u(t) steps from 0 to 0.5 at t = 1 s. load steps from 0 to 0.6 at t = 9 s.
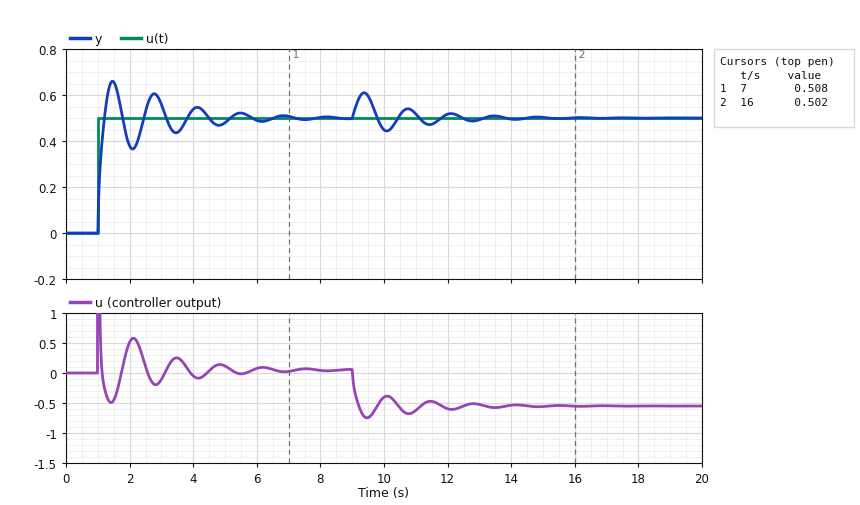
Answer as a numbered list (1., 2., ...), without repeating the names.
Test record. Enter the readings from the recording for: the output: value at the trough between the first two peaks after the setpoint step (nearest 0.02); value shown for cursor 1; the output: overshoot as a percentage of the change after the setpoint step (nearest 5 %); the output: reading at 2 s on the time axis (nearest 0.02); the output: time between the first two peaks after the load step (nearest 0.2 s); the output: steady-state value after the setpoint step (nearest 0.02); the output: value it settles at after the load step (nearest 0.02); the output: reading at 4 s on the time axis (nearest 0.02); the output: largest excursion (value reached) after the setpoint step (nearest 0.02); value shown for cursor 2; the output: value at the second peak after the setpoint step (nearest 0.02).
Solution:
1. 0.36
2. 0.508
3. 30 %
4. 0.38
5. 1.4 s
6. 0.50
7. 0.50
8. 0.54
9. 0.66
10. 0.502
11. 0.60
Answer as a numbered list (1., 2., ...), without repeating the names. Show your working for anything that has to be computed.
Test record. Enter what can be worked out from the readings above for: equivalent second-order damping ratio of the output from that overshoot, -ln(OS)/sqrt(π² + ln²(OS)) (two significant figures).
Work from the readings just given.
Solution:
1. ln(0.3) = -1.204; 1.204 / sqrt(9.870 + 1.450) = 0.36
